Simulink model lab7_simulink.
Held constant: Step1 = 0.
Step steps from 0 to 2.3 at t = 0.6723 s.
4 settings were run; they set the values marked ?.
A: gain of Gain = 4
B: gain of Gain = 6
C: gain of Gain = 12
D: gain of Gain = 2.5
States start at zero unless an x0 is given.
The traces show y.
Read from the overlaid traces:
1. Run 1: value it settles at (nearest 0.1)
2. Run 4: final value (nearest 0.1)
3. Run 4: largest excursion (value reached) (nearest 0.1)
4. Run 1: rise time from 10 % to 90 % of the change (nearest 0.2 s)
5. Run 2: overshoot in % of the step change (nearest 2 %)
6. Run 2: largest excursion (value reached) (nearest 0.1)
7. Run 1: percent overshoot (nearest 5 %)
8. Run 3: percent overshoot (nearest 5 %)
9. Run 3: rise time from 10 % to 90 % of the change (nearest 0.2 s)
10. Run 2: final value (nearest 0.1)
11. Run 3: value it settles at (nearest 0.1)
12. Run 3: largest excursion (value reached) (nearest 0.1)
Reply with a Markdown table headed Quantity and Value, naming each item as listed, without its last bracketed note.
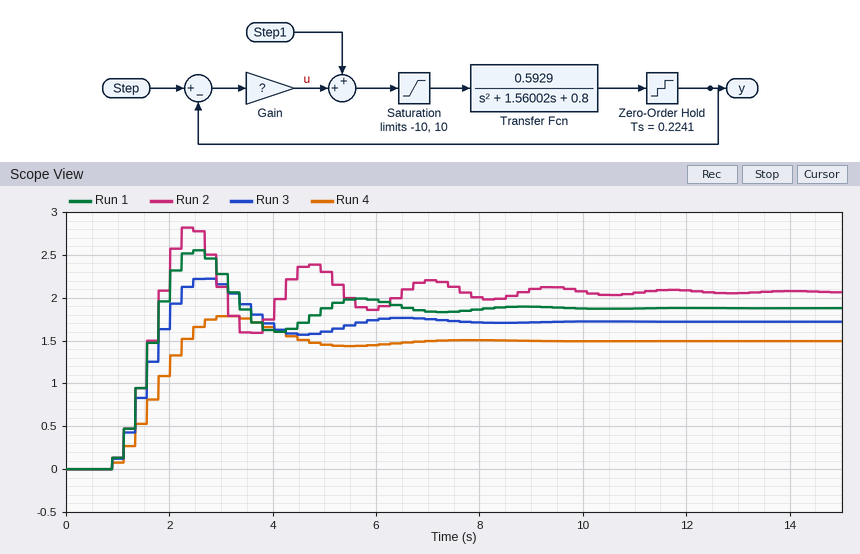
| Quantity | Value |
|---|---|
| Run 1: value it settles at | 1.9 |
| Run 4: final value | 1.5 |
| Run 4: largest excursion (value reached) | 1.8 |
| Run 1: rise time from 10 % to 90 % of the change | 0.6 s |
| Run 2: overshoot in % of the step change | 36 % |
| Run 2: largest excursion (value reached) | 2.8 |
| Run 1: percent overshoot | 35 % |
| Run 3: percent overshoot | 30 % |
| Run 3: rise time from 10 % to 90 % of the change | 0.6 s |
| Run 2: final value | 2.1 |
| Run 3: value it settles at | 1.7 |
| Run 3: largest excursion (value reached) | 2.2 |
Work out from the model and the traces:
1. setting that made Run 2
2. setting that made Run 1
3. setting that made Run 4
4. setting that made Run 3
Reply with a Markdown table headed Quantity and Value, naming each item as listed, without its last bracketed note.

| Quantity | Value |
|---|---|
| setting that made Run 2 | C |
| setting that made Run 1 | B |
| setting that made Run 4 | D |
| setting that made Run 3 | A |
